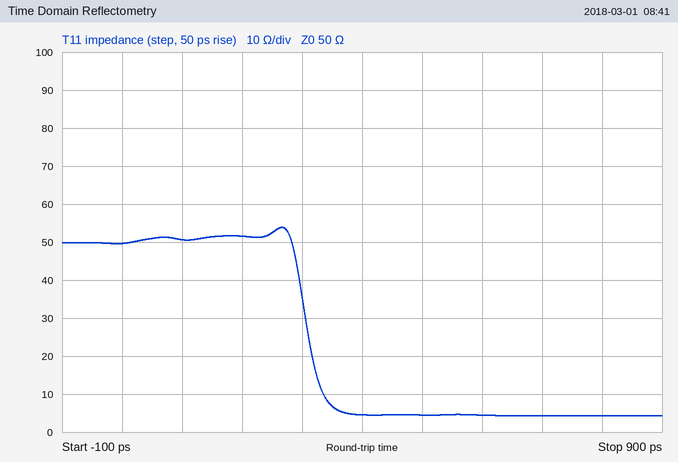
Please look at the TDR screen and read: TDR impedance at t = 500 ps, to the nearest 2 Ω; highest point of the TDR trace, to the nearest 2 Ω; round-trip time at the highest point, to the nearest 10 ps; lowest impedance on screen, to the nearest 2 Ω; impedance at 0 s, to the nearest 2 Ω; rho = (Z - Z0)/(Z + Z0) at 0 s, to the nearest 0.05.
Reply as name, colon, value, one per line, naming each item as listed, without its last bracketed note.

TDR impedance at t = 500 ps, to the nearest 2 Ω: 4 Ω
highest point of the TDR trace, to the nearest 2 Ω: 54 Ω
round-trip time at the highest point, to the nearest 10 ps: 270 ps
lowest impedance on screen, to the nearest 2 Ω: 4 Ω
impedance at 0 s, to the nearest 2 Ω: 50 Ω
rho = (Z - Z0)/(Z + Z0) at 0 s, to the nearest 0.05: 0.00
